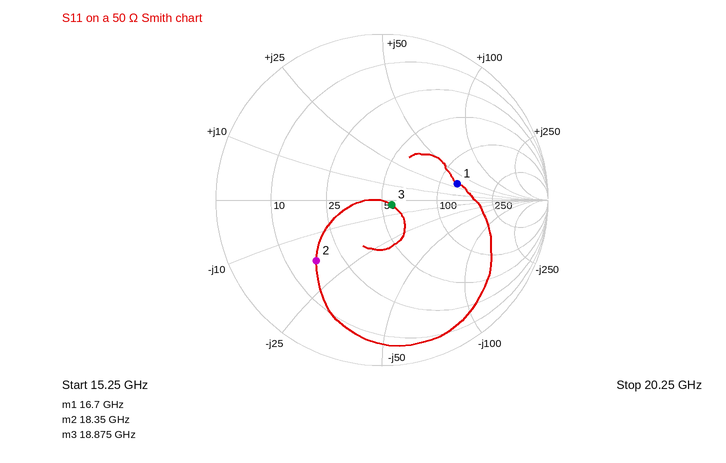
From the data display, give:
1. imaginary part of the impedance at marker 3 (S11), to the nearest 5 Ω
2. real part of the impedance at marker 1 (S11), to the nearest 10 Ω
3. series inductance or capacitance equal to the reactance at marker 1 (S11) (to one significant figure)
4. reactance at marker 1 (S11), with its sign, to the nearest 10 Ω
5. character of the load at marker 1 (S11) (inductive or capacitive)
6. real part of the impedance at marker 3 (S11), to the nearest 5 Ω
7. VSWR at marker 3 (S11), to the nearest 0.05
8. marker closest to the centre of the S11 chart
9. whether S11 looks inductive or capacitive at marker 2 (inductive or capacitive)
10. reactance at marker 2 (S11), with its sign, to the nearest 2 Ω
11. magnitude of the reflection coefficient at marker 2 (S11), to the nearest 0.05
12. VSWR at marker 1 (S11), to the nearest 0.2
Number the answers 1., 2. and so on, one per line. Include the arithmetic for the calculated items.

1. -5 Ω
2. 130 Ω
3. L = 30 Ω/(2π × 16.7 GHz) ≈ 286 pH, so 300 pH to one significant figure
4. +30 Ω
5. inductive
6. 55 Ω
7. 1.15
8. marker 3
9. capacitive
10. -18 Ω
11. 0.55
12. 2.8
